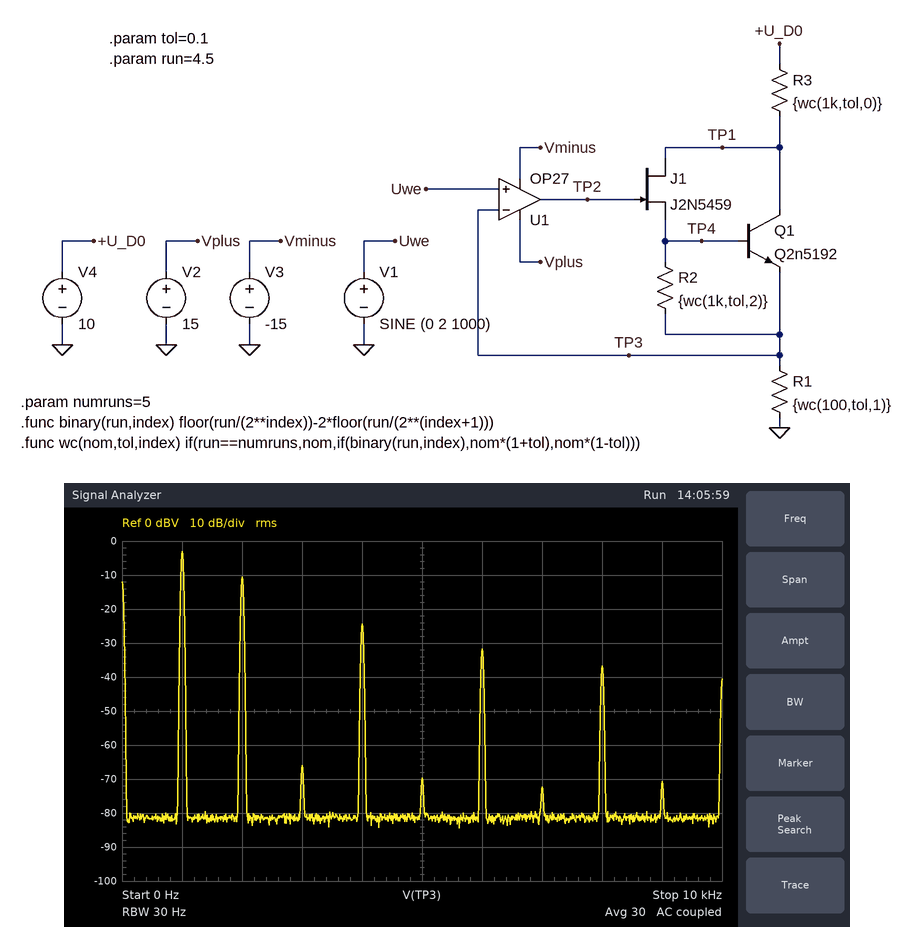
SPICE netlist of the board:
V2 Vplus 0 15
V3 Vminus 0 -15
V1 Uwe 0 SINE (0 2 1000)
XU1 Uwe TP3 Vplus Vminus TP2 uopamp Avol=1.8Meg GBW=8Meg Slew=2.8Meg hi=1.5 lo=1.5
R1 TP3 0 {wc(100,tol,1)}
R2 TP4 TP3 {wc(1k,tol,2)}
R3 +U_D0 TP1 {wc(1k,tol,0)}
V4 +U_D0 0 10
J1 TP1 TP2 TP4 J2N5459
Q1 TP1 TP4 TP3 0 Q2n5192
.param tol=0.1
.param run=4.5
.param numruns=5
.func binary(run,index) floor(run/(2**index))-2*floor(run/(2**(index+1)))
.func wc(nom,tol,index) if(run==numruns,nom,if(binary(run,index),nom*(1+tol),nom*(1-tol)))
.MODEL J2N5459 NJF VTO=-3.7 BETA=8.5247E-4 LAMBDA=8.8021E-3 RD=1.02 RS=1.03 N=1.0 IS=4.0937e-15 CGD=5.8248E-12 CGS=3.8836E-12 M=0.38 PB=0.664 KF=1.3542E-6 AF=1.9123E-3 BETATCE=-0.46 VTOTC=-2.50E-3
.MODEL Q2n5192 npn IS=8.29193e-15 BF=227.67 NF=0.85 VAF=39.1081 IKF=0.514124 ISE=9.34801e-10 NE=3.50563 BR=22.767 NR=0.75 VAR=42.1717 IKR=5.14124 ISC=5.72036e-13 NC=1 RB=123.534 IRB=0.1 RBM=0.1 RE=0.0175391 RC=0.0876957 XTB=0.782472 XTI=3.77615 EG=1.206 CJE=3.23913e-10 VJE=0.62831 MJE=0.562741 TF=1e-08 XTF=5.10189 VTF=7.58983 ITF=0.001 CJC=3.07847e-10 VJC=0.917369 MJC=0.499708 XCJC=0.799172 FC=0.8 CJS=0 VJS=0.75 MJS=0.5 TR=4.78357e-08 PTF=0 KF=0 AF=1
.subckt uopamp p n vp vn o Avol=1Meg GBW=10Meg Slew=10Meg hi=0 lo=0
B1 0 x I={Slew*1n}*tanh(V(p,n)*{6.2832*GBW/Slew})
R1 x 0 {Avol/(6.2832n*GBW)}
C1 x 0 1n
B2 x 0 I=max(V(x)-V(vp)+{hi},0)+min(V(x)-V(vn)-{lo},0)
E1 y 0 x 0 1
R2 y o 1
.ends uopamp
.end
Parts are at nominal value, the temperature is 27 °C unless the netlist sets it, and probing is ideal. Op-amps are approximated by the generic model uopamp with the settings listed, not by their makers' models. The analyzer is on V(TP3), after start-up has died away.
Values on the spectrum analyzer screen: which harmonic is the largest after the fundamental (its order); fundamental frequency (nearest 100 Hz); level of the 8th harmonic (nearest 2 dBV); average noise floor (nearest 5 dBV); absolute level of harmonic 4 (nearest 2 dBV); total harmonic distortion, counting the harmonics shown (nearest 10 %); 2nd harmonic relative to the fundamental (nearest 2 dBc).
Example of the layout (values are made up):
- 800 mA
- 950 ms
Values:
- 2
- 1.0 kHz
- -36 dBV
- -80 dBV
- -24 dBV
- 40 %
- -8 dBc
